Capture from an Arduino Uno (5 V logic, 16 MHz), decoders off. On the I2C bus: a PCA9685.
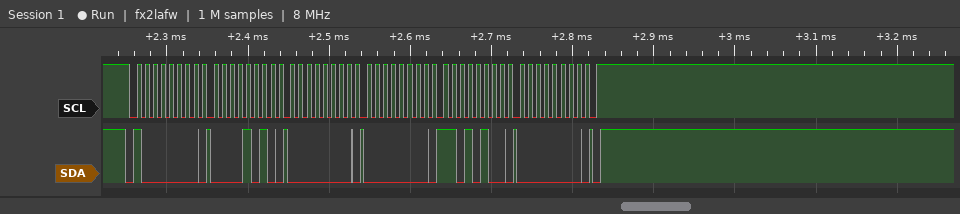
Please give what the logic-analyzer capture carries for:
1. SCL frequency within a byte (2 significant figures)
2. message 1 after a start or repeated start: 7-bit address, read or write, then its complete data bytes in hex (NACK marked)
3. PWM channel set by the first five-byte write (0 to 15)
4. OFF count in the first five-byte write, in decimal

100 kHz
0x40 write: 0A 00 00 D4 00
1
212
